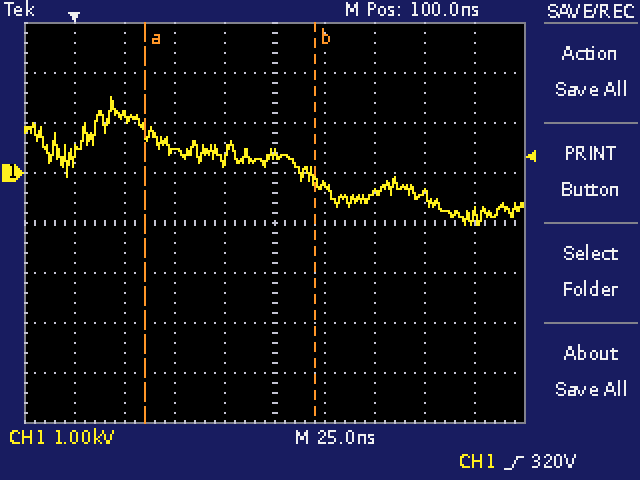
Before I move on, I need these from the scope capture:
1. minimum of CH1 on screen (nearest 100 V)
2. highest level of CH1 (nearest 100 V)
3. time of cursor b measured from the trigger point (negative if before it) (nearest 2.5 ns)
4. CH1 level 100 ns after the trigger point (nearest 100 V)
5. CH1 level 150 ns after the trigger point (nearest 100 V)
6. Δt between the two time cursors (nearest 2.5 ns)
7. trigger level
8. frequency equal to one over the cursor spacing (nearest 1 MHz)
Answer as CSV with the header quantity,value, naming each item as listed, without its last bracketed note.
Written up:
quantity,value
minimum of CH1 on screen,-1.0 kV
highest level of CH1,1.5 kV
time of cursor b measured from the trigger point (negative if before it),+120.0 ns
CH1 level 100 ns after the trigger point,400 V
CH1 level 150 ns after the trigger point,-400 V
Δt between the two time cursors,85.0 ns
trigger level,320 V
frequency equal to one over the cursor spacing,12 MHz
